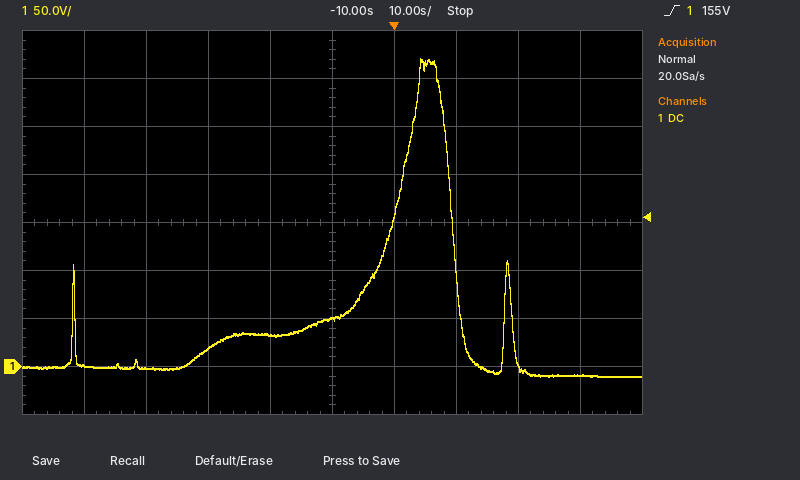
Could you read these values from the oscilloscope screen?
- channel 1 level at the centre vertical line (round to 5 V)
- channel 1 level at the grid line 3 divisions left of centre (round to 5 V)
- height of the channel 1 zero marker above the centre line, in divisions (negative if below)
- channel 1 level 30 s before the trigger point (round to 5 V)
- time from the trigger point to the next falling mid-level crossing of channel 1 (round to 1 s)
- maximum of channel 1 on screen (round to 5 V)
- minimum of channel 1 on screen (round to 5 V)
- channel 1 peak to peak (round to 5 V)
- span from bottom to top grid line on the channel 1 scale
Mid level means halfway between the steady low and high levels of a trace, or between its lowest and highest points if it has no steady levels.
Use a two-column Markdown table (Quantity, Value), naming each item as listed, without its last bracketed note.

| Quantity | Value |
|---|---|
| channel 1 level at the centre vertical line | 50 V |
| channel 1 level at the grid line 3 divisions left of centre | 0 V |
| height of the channel 1 zero marker above the centre line, in divisions | -3.0 div |
| channel 1 level 30 s before the trigger point | 20 V |
| time from the trigger point to the next falling mid-level crossing of channel 1 | 9 s |
| maximum of channel 1 on screen | 320 V |
| minimum of channel 1 on screen | -10 V |
| channel 1 peak to peak | 330 V |
| span from bottom to top grid line on the channel 1 scale | 400 V |
